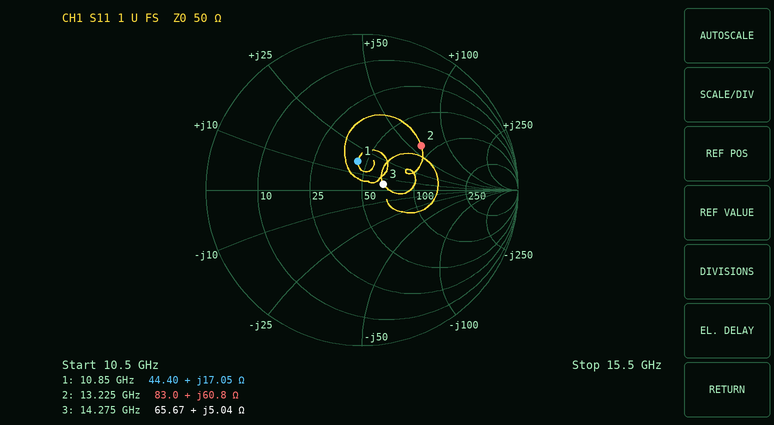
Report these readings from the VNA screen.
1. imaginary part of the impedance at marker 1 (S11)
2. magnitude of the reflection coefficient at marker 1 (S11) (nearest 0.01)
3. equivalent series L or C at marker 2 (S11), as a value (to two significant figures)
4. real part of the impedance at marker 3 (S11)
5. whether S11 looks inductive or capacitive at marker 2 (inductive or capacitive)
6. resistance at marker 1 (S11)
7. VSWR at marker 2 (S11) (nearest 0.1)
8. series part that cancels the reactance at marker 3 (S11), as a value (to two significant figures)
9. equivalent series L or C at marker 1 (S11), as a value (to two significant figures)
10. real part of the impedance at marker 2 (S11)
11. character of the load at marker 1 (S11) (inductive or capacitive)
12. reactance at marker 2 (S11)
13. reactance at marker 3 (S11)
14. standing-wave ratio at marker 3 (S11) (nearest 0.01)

+17.05 Ω
0.19
730 pH
65.67 Ω
inductive
44.40 Ω
2.8
2.2 pF
250 pH
83.0 Ω
inductive
+60.8 Ω
+5.04 Ω
1.33
